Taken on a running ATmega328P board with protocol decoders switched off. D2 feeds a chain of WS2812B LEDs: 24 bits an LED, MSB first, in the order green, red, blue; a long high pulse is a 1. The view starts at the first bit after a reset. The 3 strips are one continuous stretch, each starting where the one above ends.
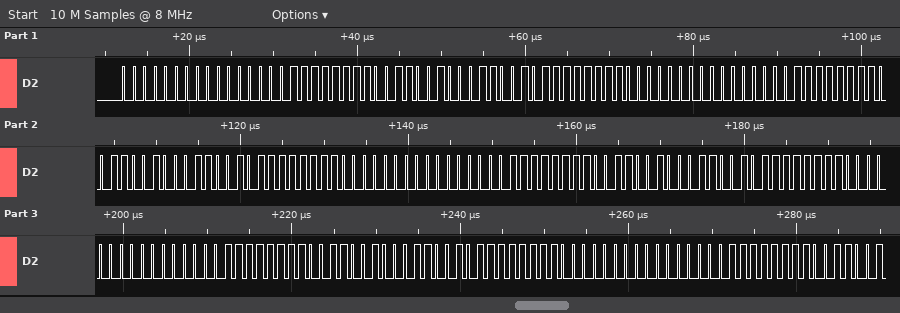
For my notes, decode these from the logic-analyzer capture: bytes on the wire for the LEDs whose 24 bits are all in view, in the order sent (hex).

00 00 FF 32 32 FF 00 00 FF 32 32 FF 00 00 FF 32 32 FF 00 00 FF 32 32 FF 00 00 FF
